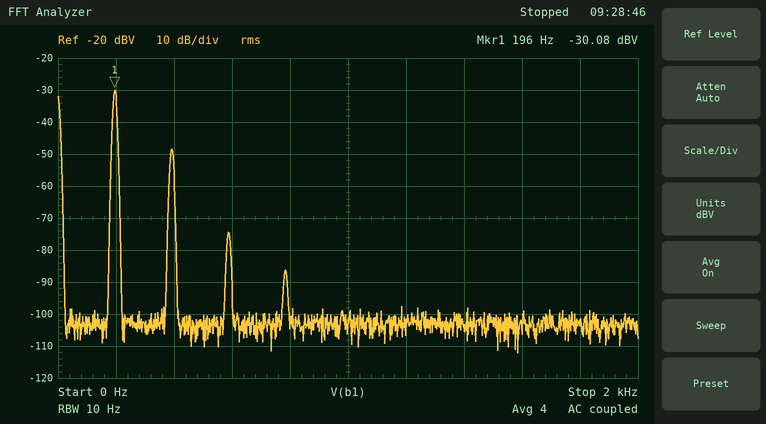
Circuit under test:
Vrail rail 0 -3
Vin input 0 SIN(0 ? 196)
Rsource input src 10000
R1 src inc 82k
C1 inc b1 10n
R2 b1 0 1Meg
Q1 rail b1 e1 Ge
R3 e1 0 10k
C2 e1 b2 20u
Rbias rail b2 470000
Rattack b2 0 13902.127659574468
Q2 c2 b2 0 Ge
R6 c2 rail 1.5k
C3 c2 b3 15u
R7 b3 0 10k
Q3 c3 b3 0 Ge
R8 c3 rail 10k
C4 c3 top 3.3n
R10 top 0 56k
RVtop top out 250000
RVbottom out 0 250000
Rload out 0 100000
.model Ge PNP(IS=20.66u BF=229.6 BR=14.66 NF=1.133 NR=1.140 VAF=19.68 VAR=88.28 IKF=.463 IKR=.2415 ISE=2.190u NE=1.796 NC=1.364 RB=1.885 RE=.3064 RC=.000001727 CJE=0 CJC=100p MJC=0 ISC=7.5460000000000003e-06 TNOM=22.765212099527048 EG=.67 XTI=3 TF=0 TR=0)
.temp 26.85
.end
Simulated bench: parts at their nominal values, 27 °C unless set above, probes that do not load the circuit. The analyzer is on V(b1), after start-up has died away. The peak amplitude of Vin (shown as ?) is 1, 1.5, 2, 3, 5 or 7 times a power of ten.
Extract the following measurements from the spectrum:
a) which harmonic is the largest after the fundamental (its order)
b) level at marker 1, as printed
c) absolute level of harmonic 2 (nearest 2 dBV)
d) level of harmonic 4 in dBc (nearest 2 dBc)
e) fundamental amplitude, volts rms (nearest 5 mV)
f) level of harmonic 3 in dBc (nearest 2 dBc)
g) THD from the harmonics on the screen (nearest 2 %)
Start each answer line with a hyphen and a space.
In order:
- 2
- -30.08 dBV
- -48 dBV
- -56 dBc
- 30 mV
- -44 dBc
- 12 %
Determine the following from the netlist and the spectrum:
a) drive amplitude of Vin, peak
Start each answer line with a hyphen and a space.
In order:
- 150 mV
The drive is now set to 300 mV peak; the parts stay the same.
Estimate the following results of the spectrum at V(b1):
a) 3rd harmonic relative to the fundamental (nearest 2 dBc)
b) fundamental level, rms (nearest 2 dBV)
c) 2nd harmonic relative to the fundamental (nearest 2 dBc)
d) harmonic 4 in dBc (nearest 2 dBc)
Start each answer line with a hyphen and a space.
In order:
- -40 dBc
- -24 dBV
- -14 dBc
- -40 dBc
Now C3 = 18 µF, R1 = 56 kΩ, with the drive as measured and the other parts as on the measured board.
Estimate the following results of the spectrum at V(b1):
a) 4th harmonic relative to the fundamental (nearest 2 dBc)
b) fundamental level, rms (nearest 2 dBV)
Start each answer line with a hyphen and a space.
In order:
- -52 dBc
- -28 dBV
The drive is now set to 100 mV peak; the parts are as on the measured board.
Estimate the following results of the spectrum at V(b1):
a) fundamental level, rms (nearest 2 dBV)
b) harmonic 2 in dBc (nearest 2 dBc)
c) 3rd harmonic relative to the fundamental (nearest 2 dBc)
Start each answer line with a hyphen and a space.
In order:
- -34 dBV
- -22 dBc
- -50 dBc
